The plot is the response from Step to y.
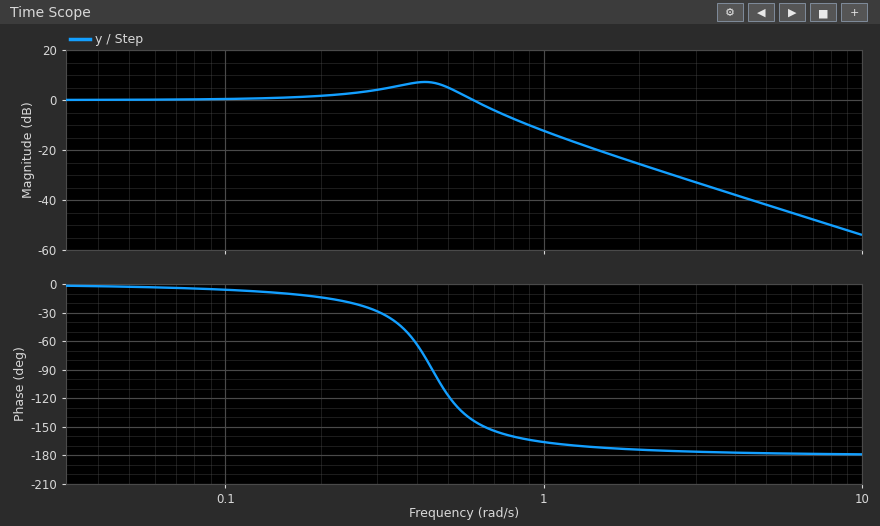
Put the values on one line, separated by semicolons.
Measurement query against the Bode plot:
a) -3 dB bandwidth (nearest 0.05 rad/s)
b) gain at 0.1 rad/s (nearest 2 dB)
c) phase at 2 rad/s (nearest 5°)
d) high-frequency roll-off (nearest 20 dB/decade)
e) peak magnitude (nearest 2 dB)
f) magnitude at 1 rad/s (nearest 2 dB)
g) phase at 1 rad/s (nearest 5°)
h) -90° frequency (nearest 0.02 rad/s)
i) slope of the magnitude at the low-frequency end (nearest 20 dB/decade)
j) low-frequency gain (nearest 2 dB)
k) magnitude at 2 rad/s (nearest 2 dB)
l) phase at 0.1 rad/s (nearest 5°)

0.65 rad/s; 0 dB; -175°; -40 dB/decade; 8 dB; -12 dB; -165°; 0.44 rad/s; 0 dB/decade; 0 dB; -26 dB; -5°
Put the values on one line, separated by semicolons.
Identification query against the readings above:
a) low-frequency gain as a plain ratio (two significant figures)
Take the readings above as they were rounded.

1.0
